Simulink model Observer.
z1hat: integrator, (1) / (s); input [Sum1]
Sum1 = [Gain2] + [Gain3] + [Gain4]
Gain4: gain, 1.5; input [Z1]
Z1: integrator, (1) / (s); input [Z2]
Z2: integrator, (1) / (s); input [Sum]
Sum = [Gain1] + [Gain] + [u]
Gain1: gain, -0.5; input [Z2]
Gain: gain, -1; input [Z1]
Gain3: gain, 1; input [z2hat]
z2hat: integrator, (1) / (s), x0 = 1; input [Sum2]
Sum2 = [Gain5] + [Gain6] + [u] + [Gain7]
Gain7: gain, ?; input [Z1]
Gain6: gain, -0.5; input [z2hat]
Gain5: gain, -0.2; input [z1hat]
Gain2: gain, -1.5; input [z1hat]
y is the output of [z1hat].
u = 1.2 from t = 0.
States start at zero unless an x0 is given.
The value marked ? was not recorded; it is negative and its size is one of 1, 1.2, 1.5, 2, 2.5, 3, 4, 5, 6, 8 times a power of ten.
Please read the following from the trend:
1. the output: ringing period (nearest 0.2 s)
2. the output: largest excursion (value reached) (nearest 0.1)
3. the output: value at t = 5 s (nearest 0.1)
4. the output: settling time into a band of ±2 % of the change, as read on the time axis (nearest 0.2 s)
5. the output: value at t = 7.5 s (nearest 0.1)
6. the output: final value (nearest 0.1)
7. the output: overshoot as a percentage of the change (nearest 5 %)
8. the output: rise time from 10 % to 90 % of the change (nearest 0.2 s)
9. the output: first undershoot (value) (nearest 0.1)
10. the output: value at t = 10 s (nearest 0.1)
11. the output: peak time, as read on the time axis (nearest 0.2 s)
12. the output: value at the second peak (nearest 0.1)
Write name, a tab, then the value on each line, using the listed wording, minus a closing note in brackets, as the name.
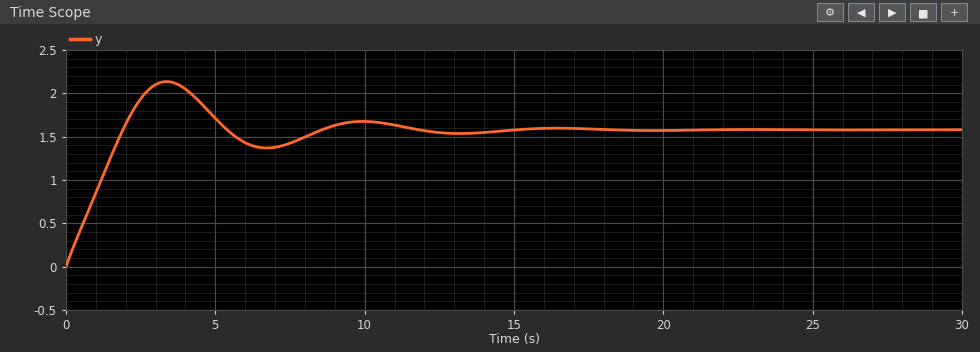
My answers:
the output: ringing period	6.6 s
the output: largest excursion (value reached)	2.1
the output: value at t = 5 s	1.7
the output: settling time into a band of ±2 % of the change, as read on the time axis	14.0 s
the output: value at t = 7.5 s	1.4
the output: final value	1.6
the output: overshoot as a percentage of the change	35 %
the output: rise time from 10 % to 90 % of the change	1.6 s
the output: first undershoot (value)	1.4
the output: value at t = 10 s	1.7
the output: peak time, as read on the time axis	3.4 s
the output: value at the second peak	1.7
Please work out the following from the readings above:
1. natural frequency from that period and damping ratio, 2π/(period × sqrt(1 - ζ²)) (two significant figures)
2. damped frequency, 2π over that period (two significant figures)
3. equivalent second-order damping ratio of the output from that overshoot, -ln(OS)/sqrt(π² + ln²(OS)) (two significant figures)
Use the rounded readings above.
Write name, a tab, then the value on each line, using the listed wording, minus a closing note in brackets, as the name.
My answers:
natural frequency from that period and damping ratio, 2π/(period × sqrt(1 - ζ²))	1.0 rad/s
damped frequency, 2π over that period	0.95 rad/s
equivalent second-order damping ratio of the output from that overshoot, -ln(OS)/sqrt(π² + ln²(OS))	0.32
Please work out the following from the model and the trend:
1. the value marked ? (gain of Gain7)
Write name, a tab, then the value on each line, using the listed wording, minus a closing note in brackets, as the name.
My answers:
the value marked ?	-0.5
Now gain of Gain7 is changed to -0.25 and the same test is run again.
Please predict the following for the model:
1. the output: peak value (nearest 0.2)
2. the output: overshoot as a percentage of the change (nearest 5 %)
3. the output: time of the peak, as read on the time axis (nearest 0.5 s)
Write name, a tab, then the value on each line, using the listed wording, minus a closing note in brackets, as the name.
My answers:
the output: peak value	2.4
the output: overshoot as a percentage of the change	25 %
the output: time of the peak, as read on the time axis	3.5 s
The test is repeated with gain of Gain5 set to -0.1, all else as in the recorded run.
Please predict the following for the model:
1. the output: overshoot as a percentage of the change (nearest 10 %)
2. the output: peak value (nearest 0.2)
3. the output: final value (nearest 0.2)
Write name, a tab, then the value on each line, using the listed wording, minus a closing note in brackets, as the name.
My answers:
the output: overshoot as a percentage of the change	30 %
the output: peak value	2.2
the output: final value	1.8
